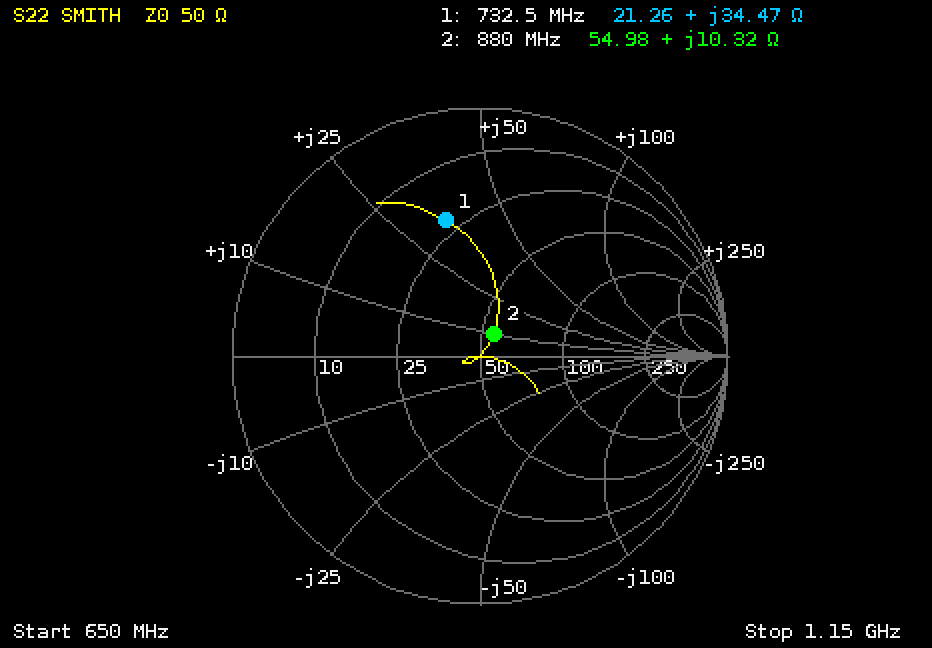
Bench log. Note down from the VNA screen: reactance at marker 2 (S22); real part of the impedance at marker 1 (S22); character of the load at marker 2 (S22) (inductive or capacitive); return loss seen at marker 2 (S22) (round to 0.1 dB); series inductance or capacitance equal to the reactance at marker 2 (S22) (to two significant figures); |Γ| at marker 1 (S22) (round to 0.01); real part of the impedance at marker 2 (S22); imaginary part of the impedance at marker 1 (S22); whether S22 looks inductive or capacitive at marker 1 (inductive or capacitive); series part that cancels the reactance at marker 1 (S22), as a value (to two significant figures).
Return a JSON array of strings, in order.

["+10.32 Ω", "21.26 Ω", "inductive", "19.3 dB", "1.9 nH", "0.57", "54.98 Ω", "+34.47 Ω", "inductive", "6.3 pF"]
